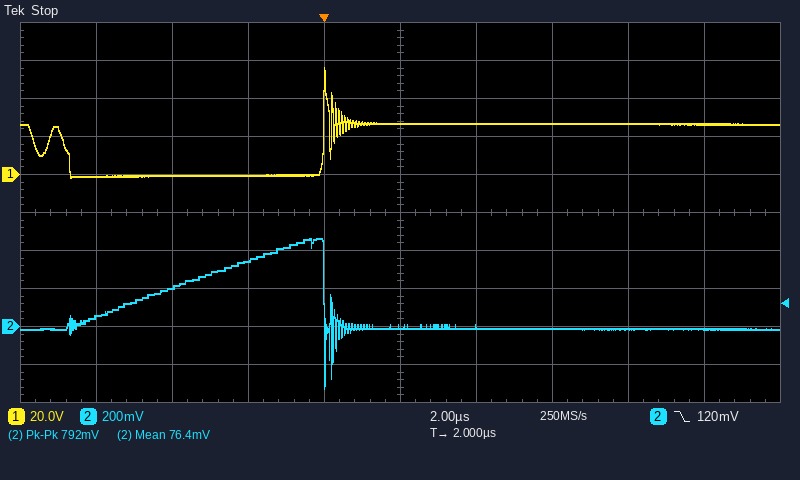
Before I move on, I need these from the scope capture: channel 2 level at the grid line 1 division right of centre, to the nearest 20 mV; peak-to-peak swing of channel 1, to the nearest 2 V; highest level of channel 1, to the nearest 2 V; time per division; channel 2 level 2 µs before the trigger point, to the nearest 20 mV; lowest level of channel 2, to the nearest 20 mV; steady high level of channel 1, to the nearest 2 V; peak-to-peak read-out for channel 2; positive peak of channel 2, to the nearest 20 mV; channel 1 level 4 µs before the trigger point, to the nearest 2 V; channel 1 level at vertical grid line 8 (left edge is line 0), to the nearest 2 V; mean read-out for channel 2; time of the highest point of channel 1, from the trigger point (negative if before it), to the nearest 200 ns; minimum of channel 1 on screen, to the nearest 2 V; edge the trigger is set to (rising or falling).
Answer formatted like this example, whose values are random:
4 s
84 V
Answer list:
0 mV
58 V
56 V
2 µs
340 mV
-320 mV
26 V
792 mV
460 mV
0 V
26 V
76.4 mV
0.0 µs
-2 V
falling
